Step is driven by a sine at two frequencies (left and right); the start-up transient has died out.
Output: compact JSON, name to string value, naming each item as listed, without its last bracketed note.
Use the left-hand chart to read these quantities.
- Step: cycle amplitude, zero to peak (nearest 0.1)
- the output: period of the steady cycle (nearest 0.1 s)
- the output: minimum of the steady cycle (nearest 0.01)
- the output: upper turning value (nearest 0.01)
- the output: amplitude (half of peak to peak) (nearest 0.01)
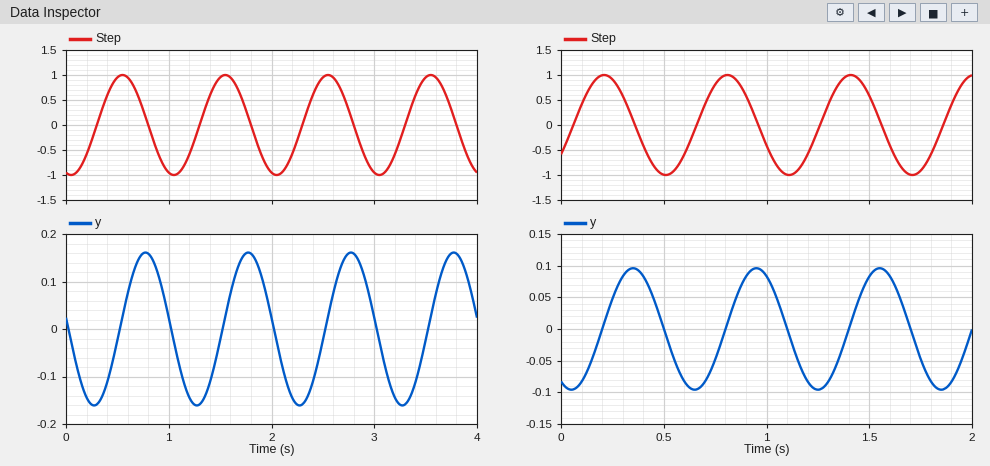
{"Step: cycle amplitude, zero to peak": "1.0", "the output: period of the steady cycle": "1.0 s", "the output: minimum of the steady cycle": "-0.16", "the output: upper turning value": "0.16", "the output: amplitude (half of peak to peak)": "0.16"}
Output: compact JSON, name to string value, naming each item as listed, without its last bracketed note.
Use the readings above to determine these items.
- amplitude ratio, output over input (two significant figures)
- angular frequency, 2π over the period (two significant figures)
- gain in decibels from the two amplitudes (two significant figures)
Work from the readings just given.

{"amplitude ratio, output over input": "0.16", "angular frequency, 2π over the period": "6.3 rad/s", "gain in decibels from the two amplitudes": "-16 dB"}
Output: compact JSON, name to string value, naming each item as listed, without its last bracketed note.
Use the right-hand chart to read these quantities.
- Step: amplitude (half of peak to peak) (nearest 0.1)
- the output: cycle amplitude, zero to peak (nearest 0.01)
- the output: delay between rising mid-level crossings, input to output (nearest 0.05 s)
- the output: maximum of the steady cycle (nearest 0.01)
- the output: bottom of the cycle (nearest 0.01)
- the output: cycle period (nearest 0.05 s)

{"Step: amplitude (half of peak to peak)": "1.0", "the output: cycle amplitude, zero to peak": "0.10", "the output: delay between rising mid-level crossings, input to output": "0.15 s", "the output: maximum of the steady cycle": "0.10", "the output: bottom of the cycle": "-0.10", "the output: cycle period": "0.60 s"}
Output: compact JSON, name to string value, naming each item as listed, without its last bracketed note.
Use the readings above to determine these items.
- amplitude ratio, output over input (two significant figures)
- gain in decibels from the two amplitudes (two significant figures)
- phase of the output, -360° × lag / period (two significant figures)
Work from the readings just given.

{"amplitude ratio, output over input": "0.10", "gain in decibels from the two amplitudes": "-20 dB", "phase of the output, -360° × lag / period": "-90°"}
